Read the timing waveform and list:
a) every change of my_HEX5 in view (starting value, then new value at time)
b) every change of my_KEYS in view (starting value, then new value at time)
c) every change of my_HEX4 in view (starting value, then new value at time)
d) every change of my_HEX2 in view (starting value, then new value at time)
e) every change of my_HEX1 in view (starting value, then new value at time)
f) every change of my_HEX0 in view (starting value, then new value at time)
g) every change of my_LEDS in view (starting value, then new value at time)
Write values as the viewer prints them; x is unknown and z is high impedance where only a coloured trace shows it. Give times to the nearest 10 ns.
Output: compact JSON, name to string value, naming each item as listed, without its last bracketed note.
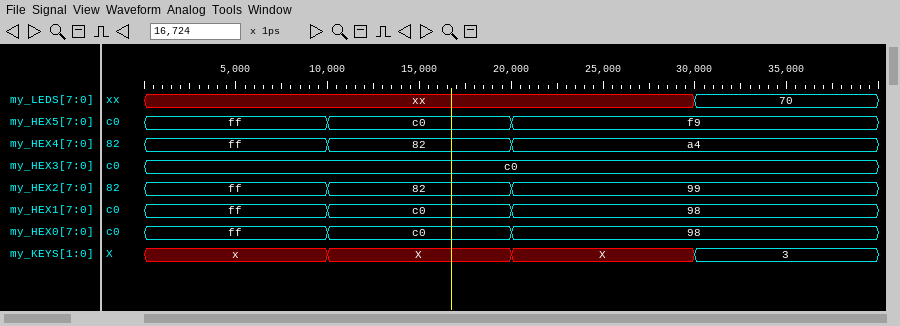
{"every change of my_HEX5 in view": "ff, c0 at 10 ns, f9 at 20 ns", "every change of my_KEYS in view": "x, X at 10 ns, X at 20 ns, 3 at 30 ns", "every change of my_HEX4 in view": "ff, 82 at 10 ns, a4 at 20 ns", "every change of my_HEX2 in view": "ff, 82 at 10 ns, 99 at 20 ns", "every change of my_HEX1 in view": "ff, c0 at 10 ns, 98 at 20 ns", "every change of my_HEX0 in view": "ff, c0 at 10 ns, 98 at 20 ns", "every change of my_LEDS in view": "xx, 70 at 30 ns"}
